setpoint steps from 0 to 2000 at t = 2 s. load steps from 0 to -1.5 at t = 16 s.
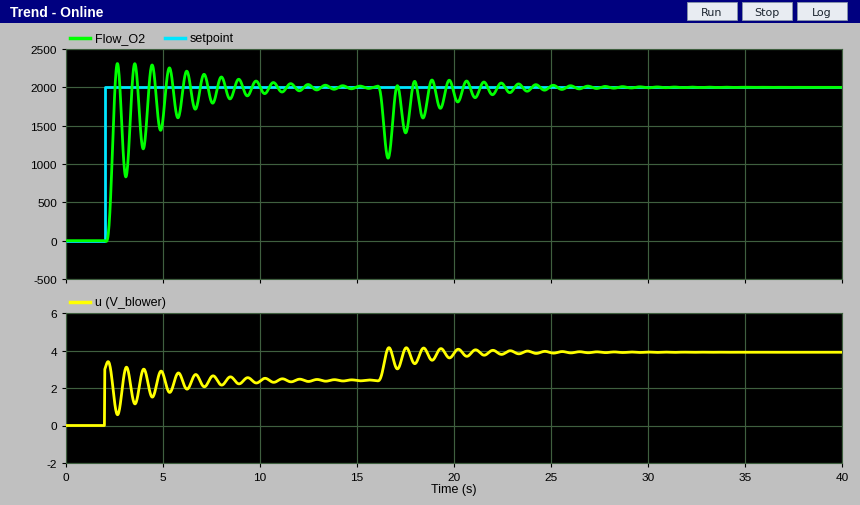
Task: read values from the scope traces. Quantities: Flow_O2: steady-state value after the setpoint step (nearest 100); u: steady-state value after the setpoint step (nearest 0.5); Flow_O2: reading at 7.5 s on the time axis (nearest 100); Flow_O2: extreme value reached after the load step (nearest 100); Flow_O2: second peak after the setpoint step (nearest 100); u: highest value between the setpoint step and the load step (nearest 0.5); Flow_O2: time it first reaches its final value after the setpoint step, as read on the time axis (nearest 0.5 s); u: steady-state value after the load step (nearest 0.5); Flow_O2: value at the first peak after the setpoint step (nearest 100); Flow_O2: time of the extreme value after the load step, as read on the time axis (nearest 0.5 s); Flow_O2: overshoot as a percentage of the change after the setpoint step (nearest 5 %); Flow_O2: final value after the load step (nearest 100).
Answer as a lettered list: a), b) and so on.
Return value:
a) 2000
b) 2.5
c) 1800
d) 1100
e) 2300
f) 3.5
g) 2.5 s
h) 4.0
i) 2300
j) 16.5 s
k) 15 %
l) 2000
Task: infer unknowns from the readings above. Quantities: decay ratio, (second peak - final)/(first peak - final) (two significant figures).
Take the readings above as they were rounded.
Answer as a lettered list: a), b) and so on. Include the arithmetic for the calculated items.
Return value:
a) (2300 - 2000) / (2300 - 2000) = 1.0
